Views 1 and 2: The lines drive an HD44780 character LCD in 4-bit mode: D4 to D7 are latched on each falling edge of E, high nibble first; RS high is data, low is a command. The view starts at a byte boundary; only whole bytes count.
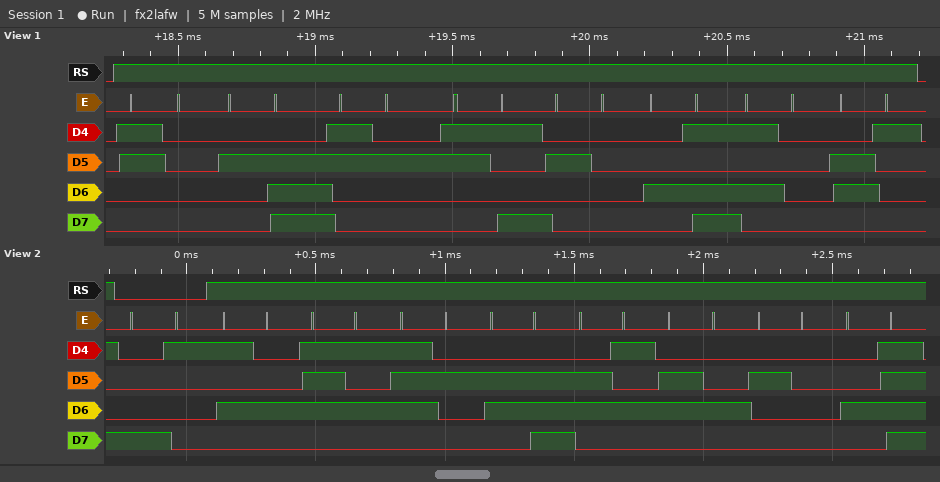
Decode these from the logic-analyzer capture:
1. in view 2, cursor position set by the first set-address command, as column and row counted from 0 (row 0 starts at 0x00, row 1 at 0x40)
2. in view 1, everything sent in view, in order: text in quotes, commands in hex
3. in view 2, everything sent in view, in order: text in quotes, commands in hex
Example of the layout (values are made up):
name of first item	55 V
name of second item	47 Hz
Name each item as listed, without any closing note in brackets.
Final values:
in view 2, cursor position set by the first set-address command, as column and row counted from 0	column 1, row 0
in view 1, everything sent in view, in order: text in quotes, commands in hex	"0.29 MPa"
in view 2, everything sent in view, in order: text in quotes, commands in hex	0x81 "Turned O"
